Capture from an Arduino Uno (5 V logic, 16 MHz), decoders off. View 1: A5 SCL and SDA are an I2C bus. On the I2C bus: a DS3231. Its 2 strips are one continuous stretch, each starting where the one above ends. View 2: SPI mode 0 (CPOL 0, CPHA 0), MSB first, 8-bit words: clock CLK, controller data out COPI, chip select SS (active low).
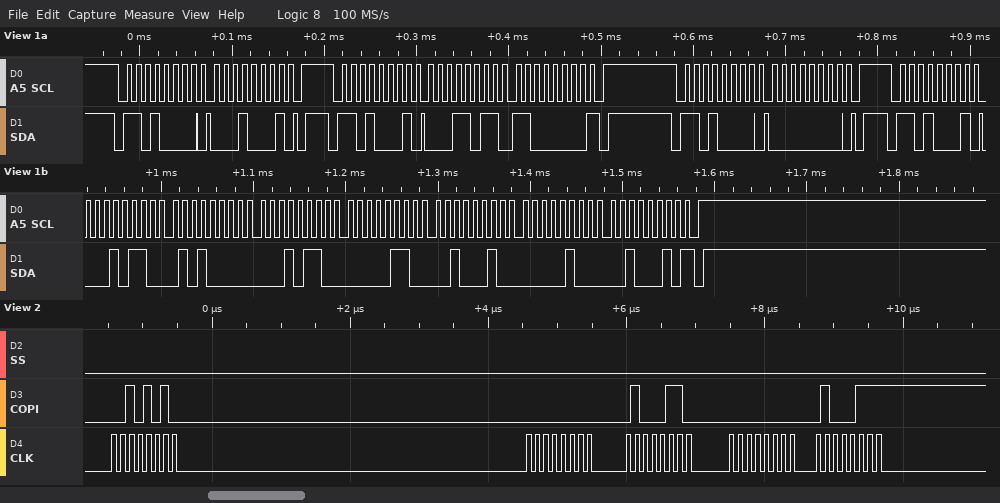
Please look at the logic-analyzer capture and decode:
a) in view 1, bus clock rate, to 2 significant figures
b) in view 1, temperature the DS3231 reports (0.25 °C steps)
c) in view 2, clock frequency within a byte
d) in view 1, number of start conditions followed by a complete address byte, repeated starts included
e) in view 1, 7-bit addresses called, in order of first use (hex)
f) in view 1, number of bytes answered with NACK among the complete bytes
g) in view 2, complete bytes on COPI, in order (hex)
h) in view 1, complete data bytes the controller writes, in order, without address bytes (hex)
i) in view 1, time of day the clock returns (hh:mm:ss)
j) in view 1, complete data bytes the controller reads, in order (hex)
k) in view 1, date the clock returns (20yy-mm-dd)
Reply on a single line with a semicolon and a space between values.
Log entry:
100 kHz; 27.75 °C; 8 MHz; 4; 0x68; 2; 2A 00 46 00 47; 11 00; 16:50:16; 1B C0 16 50 16 06 22 04 22; 2022-04-22
